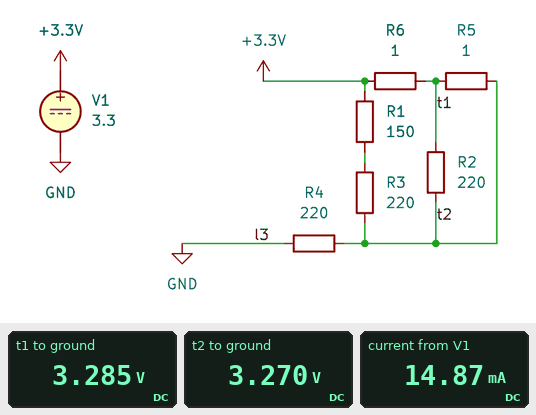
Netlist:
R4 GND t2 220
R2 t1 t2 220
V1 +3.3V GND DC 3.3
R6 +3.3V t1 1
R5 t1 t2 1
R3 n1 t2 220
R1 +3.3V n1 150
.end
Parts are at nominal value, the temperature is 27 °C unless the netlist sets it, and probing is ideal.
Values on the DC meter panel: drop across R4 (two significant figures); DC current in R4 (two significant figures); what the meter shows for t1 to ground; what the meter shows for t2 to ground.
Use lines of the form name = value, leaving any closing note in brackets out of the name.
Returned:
drop across R4 = 3.3 V
DC current in R4 = 15 mA
what the meter shows for t1 to ground = 3.285 V
what the meter shows for t2 to ground = 3.270 V
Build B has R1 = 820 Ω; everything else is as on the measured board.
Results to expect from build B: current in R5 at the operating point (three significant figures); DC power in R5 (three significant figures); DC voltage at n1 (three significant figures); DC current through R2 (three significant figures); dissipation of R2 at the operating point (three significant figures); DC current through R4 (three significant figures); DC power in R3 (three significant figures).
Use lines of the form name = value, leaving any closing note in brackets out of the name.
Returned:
current in R5 at the operating point = 14.8 mA
DC power in R5 = 218 µW
DC voltage at n1 = 3.28 V
DC current through R2 = 67.1 µA
dissipation of R2 at the operating point = 992 nW
DC current through R4 = 14.9 mA
DC power in R3 = 178 nW
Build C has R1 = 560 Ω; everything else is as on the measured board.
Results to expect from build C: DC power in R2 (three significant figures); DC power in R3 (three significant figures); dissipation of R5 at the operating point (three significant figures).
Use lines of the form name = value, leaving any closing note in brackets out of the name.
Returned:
DC power in R2 = 990 nW
DC power in R3 = 317 nW
dissipation of R5 at the operating point = 218 µW
